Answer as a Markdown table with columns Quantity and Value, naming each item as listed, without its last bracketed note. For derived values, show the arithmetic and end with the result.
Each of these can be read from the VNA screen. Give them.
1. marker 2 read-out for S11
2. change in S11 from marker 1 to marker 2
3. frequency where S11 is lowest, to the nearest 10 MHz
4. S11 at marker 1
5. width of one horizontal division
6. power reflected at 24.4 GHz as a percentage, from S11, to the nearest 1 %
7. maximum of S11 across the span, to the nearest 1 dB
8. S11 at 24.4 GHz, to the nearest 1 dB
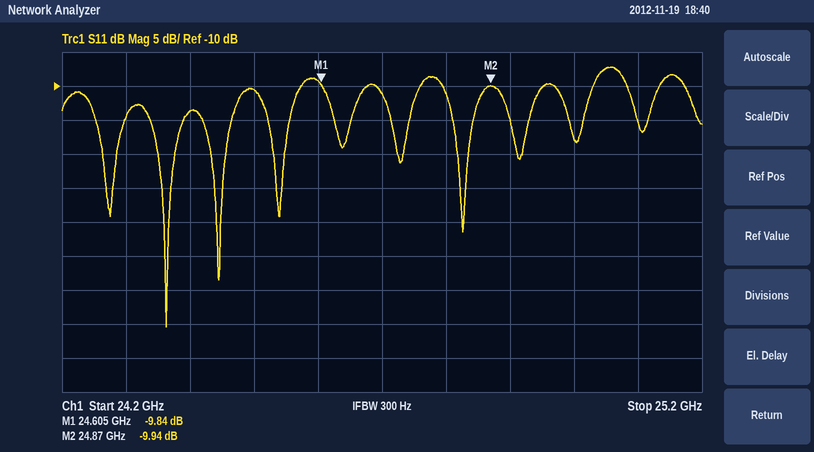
| Quantity | Value |
|---|---|
| marker 2 read-out for S11 | -9.94 dB |
| change in S11 from marker 1 to marker 2 | -9.94 − (-9.84) = -0.10 dB |
| frequency where S11 is lowest, to the nearest 10 MHz | 24.36 GHz |
| S11 at marker 1 | -9.84 dB |
| width of one horizontal division | 100 MHz |
| power reflected at 24.4 GHz as a percentage, from S11, to the nearest 1 % | 10^(-14/10) ≈ 4 % |
| maximum of S11 across the span, to the nearest 1 dB | -7 dB |
| S11 at 24.4 GHz, to the nearest 1 dB | -14 dB |
